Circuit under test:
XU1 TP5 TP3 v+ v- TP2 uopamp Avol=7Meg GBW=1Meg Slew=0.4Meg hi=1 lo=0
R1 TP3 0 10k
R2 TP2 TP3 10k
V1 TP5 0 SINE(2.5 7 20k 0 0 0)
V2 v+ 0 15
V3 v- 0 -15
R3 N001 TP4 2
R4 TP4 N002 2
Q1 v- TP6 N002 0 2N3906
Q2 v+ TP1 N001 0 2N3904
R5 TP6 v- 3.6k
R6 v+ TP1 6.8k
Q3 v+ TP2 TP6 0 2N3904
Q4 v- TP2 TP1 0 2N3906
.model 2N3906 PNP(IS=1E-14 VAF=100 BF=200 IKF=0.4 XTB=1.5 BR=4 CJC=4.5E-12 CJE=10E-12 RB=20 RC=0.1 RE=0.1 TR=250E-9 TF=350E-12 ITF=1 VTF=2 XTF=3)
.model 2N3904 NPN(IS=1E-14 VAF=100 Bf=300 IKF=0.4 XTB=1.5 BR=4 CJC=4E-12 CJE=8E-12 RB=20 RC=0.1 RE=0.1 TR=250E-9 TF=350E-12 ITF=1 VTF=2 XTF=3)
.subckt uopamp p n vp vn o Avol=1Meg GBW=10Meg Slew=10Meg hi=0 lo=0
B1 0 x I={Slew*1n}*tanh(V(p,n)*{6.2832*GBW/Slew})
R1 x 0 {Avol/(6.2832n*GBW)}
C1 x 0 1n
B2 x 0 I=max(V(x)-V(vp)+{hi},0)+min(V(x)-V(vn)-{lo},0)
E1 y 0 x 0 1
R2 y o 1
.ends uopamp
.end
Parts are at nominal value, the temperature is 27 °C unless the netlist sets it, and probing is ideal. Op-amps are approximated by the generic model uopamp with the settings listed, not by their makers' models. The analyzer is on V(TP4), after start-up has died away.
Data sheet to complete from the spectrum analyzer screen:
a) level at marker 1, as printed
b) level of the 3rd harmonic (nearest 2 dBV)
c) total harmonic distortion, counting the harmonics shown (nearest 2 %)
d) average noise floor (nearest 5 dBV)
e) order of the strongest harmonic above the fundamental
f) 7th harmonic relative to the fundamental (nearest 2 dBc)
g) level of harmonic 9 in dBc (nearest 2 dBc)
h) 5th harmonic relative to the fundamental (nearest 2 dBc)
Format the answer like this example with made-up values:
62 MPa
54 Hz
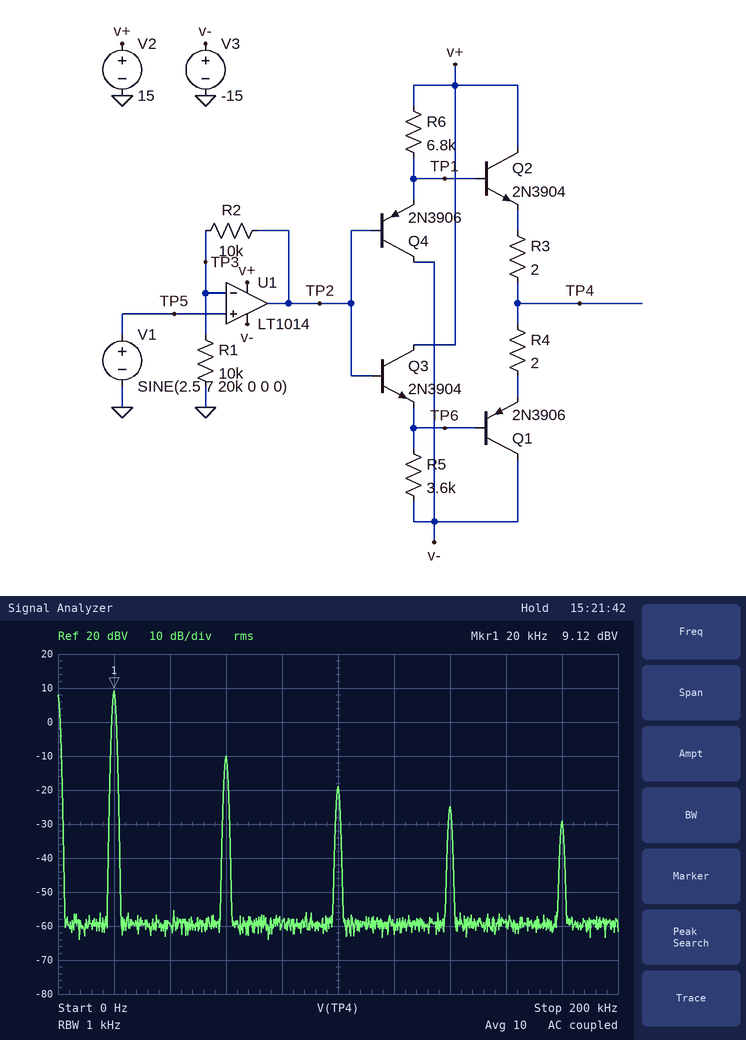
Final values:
9.12 dBV
-10 dBV
12 %
-60 dBV
3
-34 dBc
-38 dBc
-28 dBc
